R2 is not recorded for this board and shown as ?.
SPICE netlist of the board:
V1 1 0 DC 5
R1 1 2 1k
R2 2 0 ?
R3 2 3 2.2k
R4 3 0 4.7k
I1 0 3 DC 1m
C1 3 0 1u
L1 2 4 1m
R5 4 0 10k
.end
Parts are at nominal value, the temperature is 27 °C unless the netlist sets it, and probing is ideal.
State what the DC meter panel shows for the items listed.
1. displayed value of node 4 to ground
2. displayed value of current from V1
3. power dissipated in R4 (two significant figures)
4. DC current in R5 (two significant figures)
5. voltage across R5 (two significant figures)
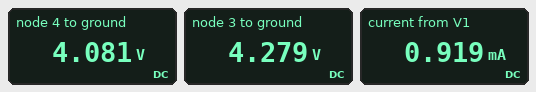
4.081 V
0.919 mA
3.9 mW
410 µA
4.1 V
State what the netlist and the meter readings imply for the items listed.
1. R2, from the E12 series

6.8 kΩ
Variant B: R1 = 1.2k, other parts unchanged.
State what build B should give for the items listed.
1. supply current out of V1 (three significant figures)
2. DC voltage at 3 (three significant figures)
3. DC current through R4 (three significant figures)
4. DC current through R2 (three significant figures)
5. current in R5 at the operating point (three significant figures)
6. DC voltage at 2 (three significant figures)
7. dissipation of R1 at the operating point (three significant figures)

870 µA
4.19 V
892 µA
582 µA
396 µA
3.96 V
908 µW
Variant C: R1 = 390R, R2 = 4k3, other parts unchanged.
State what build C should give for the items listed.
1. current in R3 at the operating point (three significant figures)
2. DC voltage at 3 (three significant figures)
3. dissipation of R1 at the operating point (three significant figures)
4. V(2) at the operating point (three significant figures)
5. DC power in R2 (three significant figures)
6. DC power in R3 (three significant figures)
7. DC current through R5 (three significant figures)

37.8 µA
4.52 V
807 µW
4.44 V
4.58 mW
3.15 µW
444 µA
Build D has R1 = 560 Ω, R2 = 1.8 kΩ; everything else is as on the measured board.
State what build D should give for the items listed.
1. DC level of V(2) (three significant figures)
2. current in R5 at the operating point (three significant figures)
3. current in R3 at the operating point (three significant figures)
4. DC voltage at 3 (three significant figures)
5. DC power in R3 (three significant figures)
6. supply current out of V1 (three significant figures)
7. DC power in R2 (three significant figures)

3.72 V
372 µA
143 µA
4.03 V
44.8 µW
2.29 mA
7.67 mW
